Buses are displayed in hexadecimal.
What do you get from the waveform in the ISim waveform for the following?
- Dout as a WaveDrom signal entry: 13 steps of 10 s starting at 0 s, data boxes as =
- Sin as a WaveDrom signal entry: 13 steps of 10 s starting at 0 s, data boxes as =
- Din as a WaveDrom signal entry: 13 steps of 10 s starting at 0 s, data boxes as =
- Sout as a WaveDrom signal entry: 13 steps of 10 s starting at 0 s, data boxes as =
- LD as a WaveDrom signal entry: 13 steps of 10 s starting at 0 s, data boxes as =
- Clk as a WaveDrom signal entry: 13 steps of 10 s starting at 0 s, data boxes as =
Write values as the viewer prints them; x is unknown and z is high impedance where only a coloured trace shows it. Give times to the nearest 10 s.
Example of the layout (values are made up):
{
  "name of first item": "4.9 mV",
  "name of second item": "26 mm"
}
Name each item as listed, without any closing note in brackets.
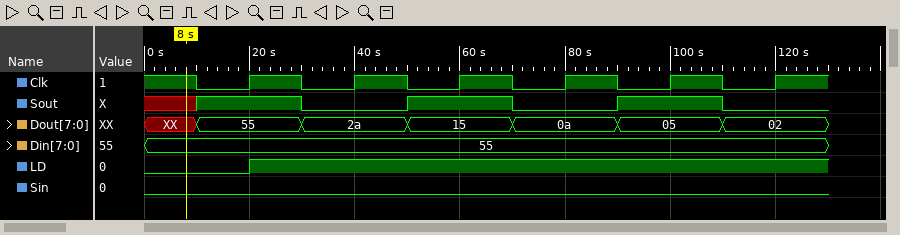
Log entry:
{
  "Dout as a WaveDrom signal entry: 13 steps of 10 s starting at 0 s, data boxes as =": "{name: 'Dout', wave: 'x=.=.=.=.=.=.', data: '55 2a 15 0a 05 02'}",
  "Sin as a WaveDrom signal entry: 13 steps of 10 s starting at 0 s, data boxes as =": "{name: 'Sin', wave: '0............'}",
  "Din as a WaveDrom signal entry: 13 steps of 10 s starting at 0 s, data boxes as =": "{name: 'Din', wave: '=............', data: '55'}",
  "Sout as a WaveDrom signal entry: 13 steps of 10 s starting at 0 s, data boxes as =": "{name: 'Sout', wave: 'x1.0.1.0.1.0.'}",
  "LD as a WaveDrom signal entry: 13 steps of 10 s starting at 0 s, data boxes as =": "{name: 'LD', wave: '0.1..........'}",
  "Clk as a WaveDrom signal entry: 13 steps of 10 s starting at 0 s, data boxes as =": "{name: 'Clk', wave: '1010101010101'}"
}
